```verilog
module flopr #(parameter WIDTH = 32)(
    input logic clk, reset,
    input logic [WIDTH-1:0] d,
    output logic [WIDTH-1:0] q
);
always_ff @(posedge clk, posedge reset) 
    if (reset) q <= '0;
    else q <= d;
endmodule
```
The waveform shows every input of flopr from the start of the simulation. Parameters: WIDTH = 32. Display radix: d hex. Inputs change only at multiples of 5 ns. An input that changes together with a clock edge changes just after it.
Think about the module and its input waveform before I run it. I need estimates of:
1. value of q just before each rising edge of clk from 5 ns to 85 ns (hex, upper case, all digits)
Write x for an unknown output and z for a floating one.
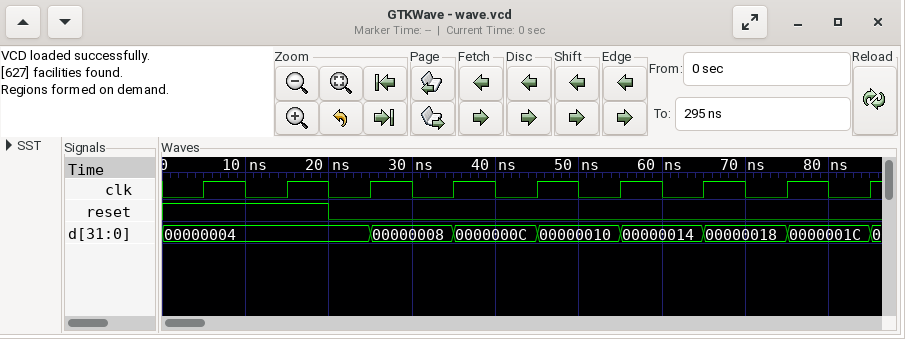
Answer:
00000000, 00000000, 00000000, 00000004, 00000008, 0000000C, 00000010, 00000014, 00000018
